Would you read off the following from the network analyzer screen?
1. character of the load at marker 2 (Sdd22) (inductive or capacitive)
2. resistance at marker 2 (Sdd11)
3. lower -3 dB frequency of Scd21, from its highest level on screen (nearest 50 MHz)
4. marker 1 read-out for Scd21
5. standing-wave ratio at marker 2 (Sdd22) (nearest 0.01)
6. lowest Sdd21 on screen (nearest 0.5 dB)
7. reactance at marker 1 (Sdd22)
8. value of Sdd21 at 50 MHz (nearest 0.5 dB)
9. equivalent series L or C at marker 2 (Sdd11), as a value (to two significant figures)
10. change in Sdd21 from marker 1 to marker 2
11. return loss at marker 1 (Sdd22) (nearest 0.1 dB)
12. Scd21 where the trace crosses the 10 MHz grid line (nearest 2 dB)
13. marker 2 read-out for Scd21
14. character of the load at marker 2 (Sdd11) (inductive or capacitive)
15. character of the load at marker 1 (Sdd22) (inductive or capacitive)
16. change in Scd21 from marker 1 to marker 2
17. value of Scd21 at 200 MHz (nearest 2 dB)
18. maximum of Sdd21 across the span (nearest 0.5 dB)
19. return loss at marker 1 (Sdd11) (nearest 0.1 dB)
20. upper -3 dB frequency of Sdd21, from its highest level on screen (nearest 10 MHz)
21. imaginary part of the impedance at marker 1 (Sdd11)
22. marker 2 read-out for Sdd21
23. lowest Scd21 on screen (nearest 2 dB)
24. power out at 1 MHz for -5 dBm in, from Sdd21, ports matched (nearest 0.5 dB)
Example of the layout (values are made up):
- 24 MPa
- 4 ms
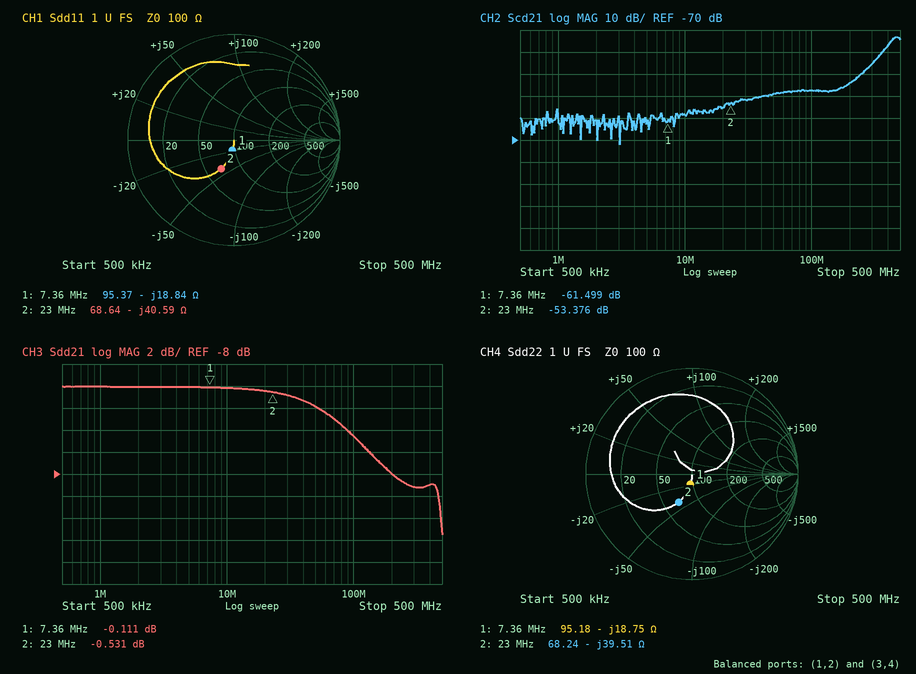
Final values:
- capacitive
- 68.64 Ω
- 400 MHz
- -61.499 dB
- 1.83
- -13.5 dB
- -18.75 Ω
- -2.0 dB
- 170 pF
- -0.420 dB
- 20.1 dB
- -58 dB
- -53.376 dB
- capacitive
- capacitive
- 8.123 dB
- -44 dB
- 0.0 dB
- 20.1 dB
- 70 MHz
- -18.84 Ω
- -0.531 dB
- -72 dB
- -5.0 dBm
